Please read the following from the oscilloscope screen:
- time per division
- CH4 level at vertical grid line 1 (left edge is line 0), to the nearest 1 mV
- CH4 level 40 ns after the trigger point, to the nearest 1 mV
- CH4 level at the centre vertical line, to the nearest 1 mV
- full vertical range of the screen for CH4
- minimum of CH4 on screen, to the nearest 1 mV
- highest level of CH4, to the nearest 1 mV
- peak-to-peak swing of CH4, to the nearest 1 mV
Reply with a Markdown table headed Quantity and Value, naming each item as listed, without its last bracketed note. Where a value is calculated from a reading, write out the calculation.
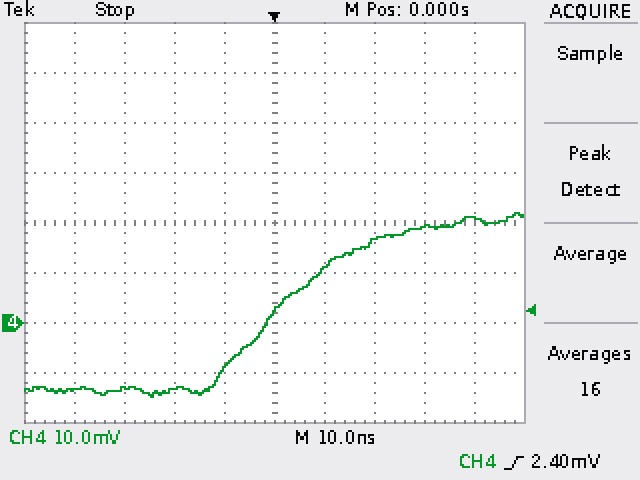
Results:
| Quantity | Value |
|---|---|
| time per division | 10 ns |
| CH4 level at vertical grid line 1 (left edge is line 0), to the nearest 1 mV | -13 mV |
| CH4 level 40 ns after the trigger point, to the nearest 1 mV | 21 mV |
| CH4 level at the centre vertical line, to the nearest 1 mV | 2 mV |
| full vertical range of the screen for CH4 | 80 mV |
| minimum of CH4 on screen, to the nearest 1 mV | -15 mV |
| highest level of CH4, to the nearest 1 mV | 22 mV |
| peak-to-peak swing of CH4, to the nearest 1 mV | 22 mV − (-15 mV) = 37 mV |
